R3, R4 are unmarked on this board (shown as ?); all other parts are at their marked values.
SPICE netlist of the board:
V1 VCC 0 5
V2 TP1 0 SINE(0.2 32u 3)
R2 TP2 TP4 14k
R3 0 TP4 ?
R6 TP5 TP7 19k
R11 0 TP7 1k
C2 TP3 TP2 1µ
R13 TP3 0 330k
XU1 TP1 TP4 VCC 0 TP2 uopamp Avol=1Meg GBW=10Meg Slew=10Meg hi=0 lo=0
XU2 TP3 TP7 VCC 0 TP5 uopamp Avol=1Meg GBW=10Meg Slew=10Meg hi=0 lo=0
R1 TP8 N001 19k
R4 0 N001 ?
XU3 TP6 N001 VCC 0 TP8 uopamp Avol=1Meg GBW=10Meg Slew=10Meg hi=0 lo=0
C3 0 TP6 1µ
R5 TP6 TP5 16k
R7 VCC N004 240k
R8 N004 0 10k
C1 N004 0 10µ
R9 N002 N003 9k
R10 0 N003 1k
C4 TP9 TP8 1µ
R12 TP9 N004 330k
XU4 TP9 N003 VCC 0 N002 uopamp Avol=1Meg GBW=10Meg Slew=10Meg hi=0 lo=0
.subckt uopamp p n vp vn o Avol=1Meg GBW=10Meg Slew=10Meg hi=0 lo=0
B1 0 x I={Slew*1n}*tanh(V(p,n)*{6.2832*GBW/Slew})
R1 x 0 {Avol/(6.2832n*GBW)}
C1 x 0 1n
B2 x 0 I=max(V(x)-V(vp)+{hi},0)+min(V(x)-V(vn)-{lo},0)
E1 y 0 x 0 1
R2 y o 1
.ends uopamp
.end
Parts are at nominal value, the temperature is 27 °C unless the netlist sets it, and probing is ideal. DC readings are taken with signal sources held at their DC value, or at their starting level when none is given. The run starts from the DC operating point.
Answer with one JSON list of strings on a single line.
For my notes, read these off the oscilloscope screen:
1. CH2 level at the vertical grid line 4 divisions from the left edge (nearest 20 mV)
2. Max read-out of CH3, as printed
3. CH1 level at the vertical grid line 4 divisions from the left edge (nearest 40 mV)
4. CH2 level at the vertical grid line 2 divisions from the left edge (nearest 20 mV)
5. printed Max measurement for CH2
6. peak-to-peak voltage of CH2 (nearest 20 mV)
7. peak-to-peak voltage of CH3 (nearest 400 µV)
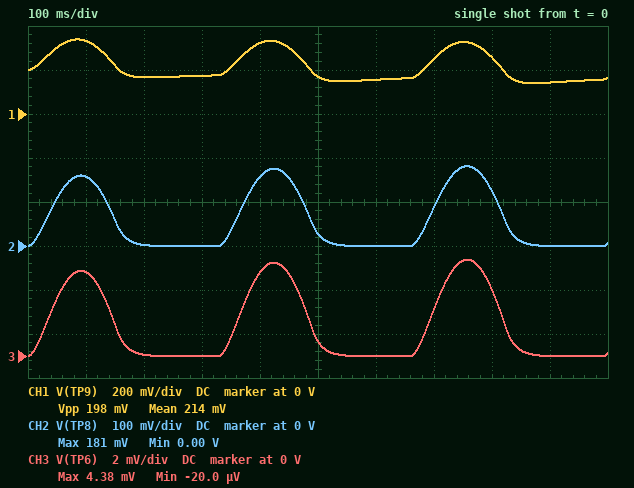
["160 mV", "4.38 mV", "320 mV", "0 V", "181 mV", "180 mV", "4.4 mV"]
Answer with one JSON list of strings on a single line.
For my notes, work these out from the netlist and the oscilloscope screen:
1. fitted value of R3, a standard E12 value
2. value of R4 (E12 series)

["2.2 kΩ", "470 Ω"]
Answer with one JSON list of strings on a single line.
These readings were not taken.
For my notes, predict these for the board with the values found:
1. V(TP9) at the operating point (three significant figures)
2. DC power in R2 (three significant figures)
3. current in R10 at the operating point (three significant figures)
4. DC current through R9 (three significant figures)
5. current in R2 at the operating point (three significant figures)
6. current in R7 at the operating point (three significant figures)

["200 mV", "116 µW", "200 µA", "200 µA", "90.9 µA", "20.0 µA"]
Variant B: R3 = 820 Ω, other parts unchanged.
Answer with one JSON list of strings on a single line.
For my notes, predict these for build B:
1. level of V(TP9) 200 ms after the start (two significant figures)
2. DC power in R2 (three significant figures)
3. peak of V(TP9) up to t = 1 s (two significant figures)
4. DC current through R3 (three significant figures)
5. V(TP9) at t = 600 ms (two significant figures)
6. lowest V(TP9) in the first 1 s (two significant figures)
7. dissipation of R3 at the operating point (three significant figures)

["120 mV", "833 µW", "540 mV", "244 µA", "92 mV", "54 mV", "48.8 µW"]
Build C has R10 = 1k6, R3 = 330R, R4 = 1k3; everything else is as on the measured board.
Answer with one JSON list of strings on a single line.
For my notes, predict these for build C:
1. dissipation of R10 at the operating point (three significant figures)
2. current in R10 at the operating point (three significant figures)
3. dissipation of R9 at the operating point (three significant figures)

["25.0 µW", "125 µA", "141 µW"]
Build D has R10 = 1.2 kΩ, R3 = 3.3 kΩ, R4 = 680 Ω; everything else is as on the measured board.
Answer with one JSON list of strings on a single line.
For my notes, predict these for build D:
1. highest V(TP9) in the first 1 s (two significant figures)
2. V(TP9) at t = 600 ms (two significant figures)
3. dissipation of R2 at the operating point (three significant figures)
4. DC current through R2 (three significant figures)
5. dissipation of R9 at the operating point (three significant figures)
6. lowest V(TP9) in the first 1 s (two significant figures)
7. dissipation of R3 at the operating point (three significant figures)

["270 mV", "180 mV", "51.4 µW", "60.6 µA", "250 µW", "170 mV", "12.1 µW"]
